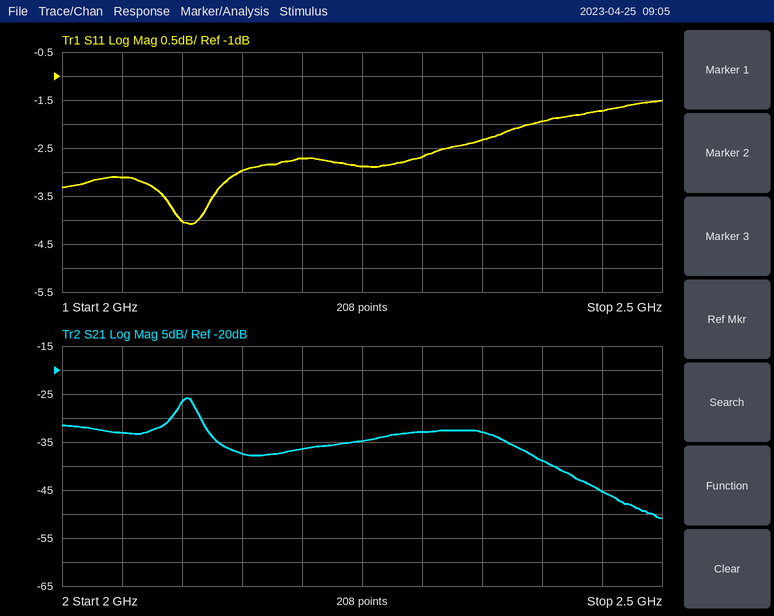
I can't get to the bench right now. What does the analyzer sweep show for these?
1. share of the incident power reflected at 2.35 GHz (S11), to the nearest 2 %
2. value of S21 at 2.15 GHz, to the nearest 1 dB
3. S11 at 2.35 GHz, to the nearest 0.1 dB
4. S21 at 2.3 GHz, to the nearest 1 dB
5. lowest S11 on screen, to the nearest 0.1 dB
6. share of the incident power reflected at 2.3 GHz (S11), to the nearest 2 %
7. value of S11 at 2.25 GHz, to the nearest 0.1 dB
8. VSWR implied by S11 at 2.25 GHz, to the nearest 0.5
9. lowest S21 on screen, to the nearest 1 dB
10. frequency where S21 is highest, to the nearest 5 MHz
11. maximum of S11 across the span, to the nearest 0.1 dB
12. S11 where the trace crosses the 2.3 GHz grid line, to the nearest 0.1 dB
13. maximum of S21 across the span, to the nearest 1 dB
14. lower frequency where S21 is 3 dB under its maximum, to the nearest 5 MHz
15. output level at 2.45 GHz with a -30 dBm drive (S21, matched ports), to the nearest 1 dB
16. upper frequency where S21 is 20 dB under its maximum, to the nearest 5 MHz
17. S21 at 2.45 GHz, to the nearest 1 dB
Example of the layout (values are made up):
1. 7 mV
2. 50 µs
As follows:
1. 58 %
2. -37 dB
3. -2.3 dB
4. -33 dB
5. -4.1 dB
6. 54 %
7. -2.9 dB
8. 6.0
9. -51 dB
10. 2.105 GHz
11. -1.5 dB
12. -2.7 dB
13. -26 dB
14. 2.095 GHz
15. -75 dBm
16. 2.455 GHz
17. -45 dB
